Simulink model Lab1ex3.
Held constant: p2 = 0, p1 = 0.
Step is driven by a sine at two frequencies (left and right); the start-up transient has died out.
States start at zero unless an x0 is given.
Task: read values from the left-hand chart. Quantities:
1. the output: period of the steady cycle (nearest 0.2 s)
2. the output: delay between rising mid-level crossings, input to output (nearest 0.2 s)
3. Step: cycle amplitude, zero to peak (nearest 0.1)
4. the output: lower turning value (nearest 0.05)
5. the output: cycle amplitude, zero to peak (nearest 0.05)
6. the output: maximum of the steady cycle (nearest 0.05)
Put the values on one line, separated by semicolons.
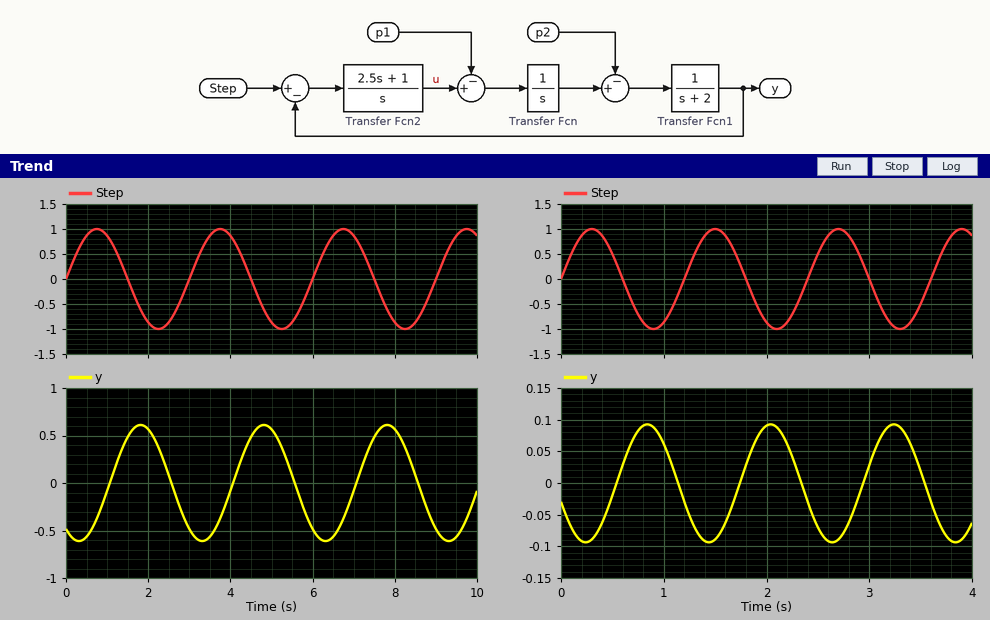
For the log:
3.0 s; 1.0 s; 1.0; -0.60; 0.60; 0.60
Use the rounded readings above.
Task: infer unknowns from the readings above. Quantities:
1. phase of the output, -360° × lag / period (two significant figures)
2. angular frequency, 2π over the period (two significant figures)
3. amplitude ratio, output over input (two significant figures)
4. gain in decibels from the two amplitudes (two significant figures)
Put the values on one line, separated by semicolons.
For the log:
-120°; 2.1 rad/s; 0.60; -4.4 dB
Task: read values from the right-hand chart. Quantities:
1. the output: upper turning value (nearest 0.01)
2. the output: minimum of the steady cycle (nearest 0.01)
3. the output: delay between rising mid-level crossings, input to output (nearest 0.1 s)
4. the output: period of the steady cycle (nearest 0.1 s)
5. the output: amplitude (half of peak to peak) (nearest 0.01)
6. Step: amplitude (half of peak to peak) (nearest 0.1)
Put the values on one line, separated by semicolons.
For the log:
0.09; -0.09; 0.5 s; 1.2 s; 0.09; 1.0
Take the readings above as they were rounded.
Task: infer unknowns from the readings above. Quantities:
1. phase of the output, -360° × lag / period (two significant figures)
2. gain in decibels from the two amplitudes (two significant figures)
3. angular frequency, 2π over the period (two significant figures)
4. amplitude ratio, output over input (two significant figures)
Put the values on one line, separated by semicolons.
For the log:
-150°; -21 dB; 5.2 rad/s; 0.090
